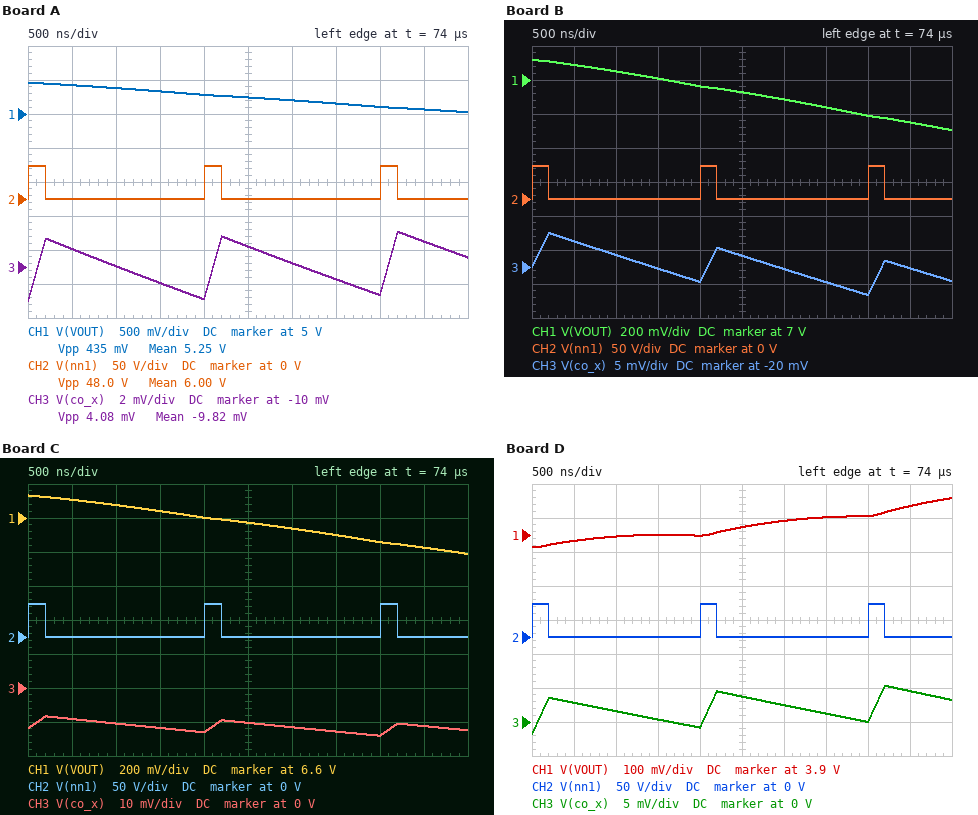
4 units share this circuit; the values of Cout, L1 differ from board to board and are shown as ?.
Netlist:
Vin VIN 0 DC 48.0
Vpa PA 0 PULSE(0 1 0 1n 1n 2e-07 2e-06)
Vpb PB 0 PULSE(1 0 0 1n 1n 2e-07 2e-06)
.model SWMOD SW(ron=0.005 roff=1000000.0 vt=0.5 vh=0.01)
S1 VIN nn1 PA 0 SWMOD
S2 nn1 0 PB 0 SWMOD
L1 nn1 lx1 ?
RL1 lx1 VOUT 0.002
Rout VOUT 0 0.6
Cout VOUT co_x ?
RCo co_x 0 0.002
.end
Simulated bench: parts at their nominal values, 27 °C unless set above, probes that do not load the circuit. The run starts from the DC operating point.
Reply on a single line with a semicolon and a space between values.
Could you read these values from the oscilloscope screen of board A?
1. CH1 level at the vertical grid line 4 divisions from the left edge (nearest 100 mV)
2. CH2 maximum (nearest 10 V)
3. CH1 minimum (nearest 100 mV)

5.3 V; 50 V; 5.0 V
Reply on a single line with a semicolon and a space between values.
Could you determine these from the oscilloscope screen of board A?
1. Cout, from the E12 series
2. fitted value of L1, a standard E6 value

56 µF; 4.7 µH
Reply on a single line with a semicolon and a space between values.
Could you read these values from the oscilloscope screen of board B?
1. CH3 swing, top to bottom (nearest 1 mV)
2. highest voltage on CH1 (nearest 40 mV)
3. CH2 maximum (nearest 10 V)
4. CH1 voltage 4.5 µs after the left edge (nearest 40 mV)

9 mV; 7.12 V; 50 V; 6.76 V
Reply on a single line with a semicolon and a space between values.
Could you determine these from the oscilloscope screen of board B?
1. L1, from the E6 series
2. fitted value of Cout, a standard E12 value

3.3 µH; 120 µF
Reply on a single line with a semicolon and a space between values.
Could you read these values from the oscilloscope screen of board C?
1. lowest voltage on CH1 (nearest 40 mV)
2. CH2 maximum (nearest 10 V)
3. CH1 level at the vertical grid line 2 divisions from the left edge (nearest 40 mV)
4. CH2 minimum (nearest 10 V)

6.40 V; 50 V; 6.68 V; 0 V
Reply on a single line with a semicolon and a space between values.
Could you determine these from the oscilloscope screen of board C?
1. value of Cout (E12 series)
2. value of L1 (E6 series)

82 µF; 4.7 µH
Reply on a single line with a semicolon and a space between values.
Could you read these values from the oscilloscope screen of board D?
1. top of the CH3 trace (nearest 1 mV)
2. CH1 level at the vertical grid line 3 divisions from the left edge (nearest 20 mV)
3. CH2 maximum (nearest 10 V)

5 mV; 3.90 V; 50 V
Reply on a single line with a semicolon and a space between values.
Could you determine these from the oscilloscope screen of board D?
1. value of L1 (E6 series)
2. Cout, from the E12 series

3.3 µH; 39 µF
